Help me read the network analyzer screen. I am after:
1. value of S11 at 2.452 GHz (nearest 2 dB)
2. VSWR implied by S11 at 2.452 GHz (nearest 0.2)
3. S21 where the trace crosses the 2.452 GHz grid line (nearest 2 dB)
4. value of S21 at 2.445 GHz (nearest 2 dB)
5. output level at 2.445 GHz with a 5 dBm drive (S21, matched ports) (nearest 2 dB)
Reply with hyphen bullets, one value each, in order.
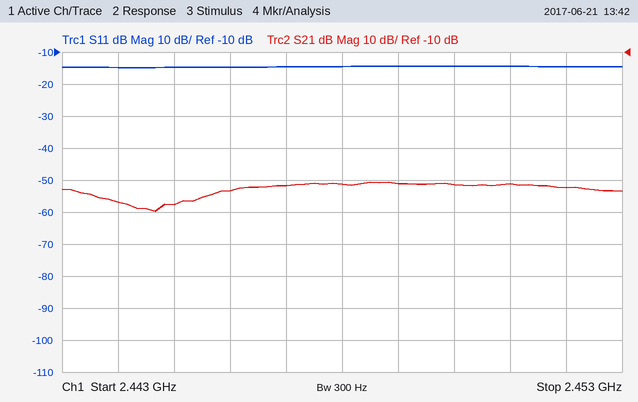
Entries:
- -14 dB
- 1.4
- -52 dB
- -58 dB
- -52 dBm
